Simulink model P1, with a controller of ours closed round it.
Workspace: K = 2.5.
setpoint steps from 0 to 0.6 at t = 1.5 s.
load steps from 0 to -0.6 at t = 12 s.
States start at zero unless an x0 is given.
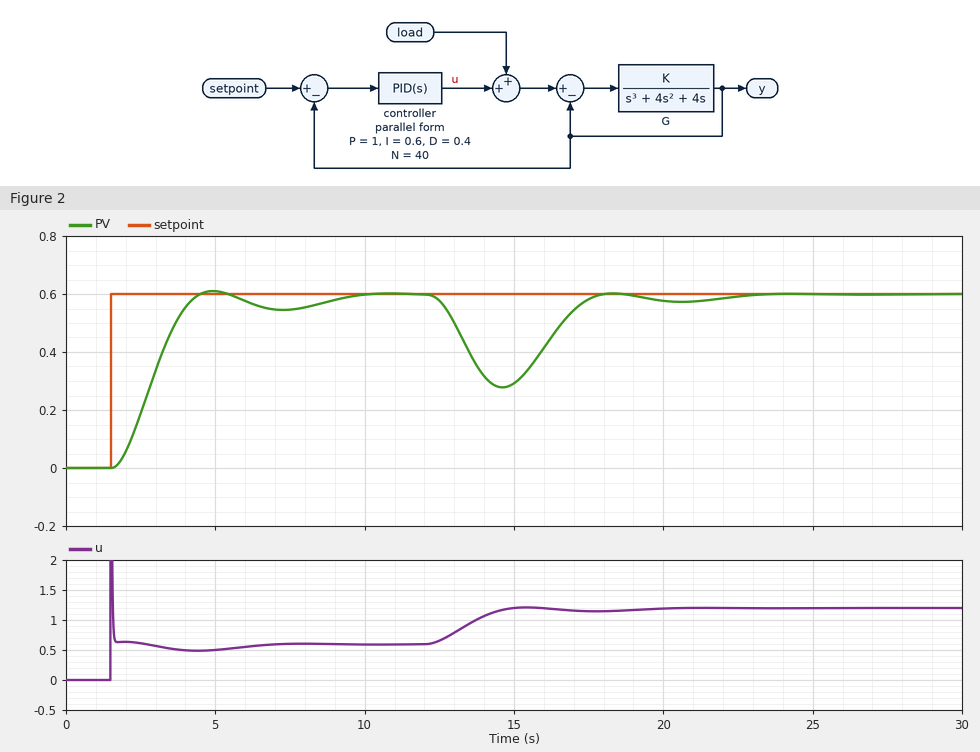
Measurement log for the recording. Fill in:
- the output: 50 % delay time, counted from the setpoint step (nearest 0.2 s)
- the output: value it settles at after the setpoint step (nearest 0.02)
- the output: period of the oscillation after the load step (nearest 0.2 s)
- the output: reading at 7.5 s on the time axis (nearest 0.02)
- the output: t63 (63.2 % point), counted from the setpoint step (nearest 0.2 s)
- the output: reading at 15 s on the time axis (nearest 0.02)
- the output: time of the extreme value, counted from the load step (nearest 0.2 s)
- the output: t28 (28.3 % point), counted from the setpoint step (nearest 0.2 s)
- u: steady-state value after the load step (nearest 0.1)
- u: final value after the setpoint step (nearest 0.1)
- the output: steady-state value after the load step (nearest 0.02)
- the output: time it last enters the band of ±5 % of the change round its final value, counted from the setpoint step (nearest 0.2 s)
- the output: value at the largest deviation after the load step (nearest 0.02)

1.4 s
0.60
6.0 s
0.54
1.6 s
0.30
2.6 s
1.0 s
1.2
0.6
0.60
7.2 s
0.28
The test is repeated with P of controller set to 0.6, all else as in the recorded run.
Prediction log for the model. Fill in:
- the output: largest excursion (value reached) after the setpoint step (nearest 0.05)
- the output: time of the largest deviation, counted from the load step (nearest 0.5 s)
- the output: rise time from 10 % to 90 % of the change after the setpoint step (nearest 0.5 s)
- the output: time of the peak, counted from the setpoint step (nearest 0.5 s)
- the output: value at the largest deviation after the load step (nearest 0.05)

0.65
3.0 s
2.5 s
4.5 s
0.25
